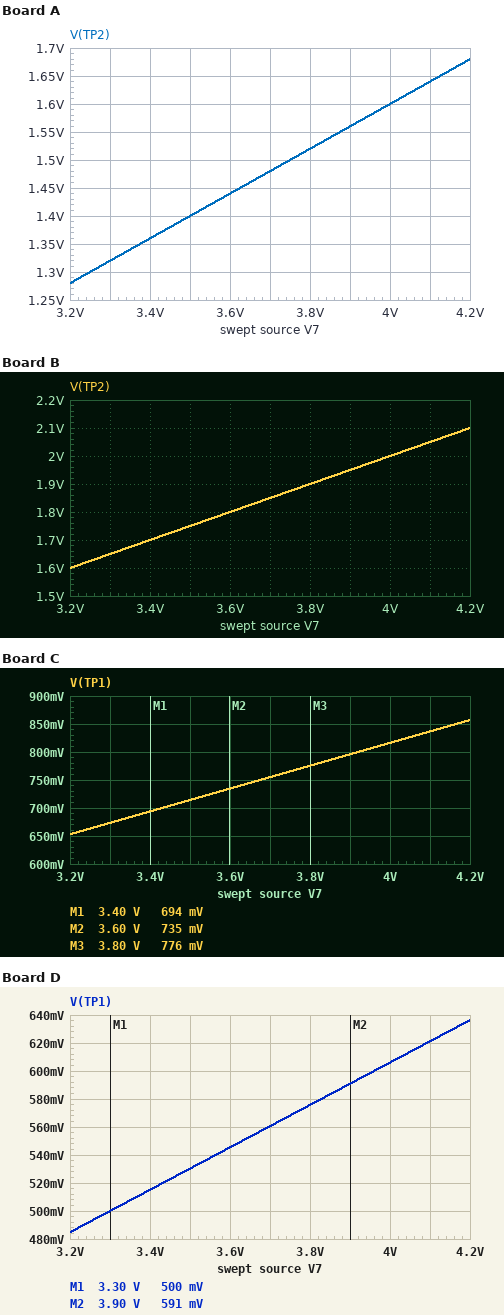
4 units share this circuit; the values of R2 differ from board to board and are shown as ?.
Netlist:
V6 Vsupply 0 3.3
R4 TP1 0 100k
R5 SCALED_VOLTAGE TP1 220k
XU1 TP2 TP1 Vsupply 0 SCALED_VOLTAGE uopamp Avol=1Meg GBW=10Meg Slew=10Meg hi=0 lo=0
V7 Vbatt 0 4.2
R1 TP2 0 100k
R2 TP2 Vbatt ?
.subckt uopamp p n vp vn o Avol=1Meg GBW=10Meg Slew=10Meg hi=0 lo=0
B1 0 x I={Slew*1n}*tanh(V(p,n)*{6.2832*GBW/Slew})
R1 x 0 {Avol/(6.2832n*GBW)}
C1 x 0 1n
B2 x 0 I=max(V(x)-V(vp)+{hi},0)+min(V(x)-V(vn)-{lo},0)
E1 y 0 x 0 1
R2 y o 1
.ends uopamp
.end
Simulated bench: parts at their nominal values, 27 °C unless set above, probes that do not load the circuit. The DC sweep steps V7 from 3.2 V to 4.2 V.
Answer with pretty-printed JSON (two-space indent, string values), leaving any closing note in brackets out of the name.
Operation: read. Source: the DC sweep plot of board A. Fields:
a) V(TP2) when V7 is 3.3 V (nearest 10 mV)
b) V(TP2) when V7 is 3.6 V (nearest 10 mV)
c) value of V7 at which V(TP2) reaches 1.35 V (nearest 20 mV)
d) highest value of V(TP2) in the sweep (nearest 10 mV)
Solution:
{
  "V(TP2) when V7 is 3.3 V": "1.32 V",
  "V(TP2) when V7 is 3.6 V": "1.44 V",
  "value of V7 at which V(TP2) reaches 1.35 V": "3.38 V",
  "highest value of V(TP2) in the sweep": "1.68 V"
}
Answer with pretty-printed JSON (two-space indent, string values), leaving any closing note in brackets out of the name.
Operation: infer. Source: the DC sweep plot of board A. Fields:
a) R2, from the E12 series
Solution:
{
  "R2, from the E12 series": "150 kΩ"
}
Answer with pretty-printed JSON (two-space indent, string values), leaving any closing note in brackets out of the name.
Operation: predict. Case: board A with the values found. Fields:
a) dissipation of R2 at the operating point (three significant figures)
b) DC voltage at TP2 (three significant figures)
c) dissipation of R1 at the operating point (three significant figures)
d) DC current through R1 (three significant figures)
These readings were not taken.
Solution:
{
  "dissipation of R2 at the operating point": "42.3 µW",
  "DC voltage at TP2": "1.68 V",
  "dissipation of R1 at the operating point": "28.2 µW",
  "DC current through R1": "16.8 µA"
}
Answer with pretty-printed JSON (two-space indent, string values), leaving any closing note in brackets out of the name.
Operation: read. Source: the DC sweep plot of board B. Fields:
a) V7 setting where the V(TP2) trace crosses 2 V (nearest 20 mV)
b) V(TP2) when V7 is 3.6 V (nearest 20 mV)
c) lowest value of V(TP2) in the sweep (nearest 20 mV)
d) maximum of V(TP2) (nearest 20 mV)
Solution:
{
  "V7 setting where the V(TP2) trace crosses 2 V": "4.00 V",
  "V(TP2) when V7 is 3.6 V": "1.80 V",
  "lowest value of V(TP2) in the sweep": "1.60 V",
  "maximum of V(TP2)": "2.10 V"
}
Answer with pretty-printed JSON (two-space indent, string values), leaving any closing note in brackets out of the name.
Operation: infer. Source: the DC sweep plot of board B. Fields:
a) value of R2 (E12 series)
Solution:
{
  "value of R2": "100 kΩ"
}
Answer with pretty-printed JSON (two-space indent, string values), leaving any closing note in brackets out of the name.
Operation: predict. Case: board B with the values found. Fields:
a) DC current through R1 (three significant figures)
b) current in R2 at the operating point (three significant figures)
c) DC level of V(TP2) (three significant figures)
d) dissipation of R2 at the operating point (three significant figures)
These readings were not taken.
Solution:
{
  "DC current through R1": "21.0 µA",
  "current in R2 at the operating point": "21.0 µA",
  "DC level of V(TP2)": "2.10 V",
  "dissipation of R2 at the operating point": "44.1 µW"
}
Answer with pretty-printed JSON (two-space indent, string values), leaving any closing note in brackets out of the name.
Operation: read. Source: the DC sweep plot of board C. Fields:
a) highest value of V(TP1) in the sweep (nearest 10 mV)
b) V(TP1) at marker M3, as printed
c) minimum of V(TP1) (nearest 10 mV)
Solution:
{
  "highest value of V(TP1) in the sweep": "860 mV",
  "V(TP1) at marker M3, as printed": "776 mV",
  "minimum of V(TP1)": "650 mV"
}
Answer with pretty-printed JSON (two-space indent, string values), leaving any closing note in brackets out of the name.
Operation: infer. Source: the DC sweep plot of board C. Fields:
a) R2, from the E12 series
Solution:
{
  "R2, from the E12 series": "390 kΩ"
}
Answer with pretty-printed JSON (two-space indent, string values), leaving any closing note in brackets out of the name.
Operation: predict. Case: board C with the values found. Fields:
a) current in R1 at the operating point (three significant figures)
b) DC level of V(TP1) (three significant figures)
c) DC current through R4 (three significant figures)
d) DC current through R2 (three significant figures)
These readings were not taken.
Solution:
{
  "current in R1 at the operating point": "8.57 µA",
  "DC level of V(TP1)": "857 mV",
  "DC current through R4": "8.57 µA",
  "DC current through R2": "8.57 µA"
}
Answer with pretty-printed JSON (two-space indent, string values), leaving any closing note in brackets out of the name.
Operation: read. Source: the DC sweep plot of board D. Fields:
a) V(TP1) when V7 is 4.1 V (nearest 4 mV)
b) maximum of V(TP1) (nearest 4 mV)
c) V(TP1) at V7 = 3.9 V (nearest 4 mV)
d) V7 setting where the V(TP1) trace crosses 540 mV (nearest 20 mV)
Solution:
{
  "V(TP1) when V7 is 4.1 V": "620 mV",
  "maximum of V(TP1)": "636 mV",
  "V(TP1) at V7 = 3.9 V": "592 mV",
  "V7 setting where the V(TP1) trace crosses 540 mV": "3.56 V"
}
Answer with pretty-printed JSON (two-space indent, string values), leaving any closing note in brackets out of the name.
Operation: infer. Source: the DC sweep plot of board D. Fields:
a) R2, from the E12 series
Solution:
{
  "R2, from the E12 series": "560 kΩ"
}
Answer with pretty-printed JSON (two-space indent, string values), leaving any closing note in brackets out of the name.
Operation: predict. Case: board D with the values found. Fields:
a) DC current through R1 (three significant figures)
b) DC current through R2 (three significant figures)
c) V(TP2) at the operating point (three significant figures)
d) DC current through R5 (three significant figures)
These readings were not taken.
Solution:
{
  "DC current through R1": "6.36 µA",
  "DC current through R2": "6.36 µA",
  "V(TP2) at the operating point": "636 mV",
  "DC current through R5": "6.36 µA"
}
